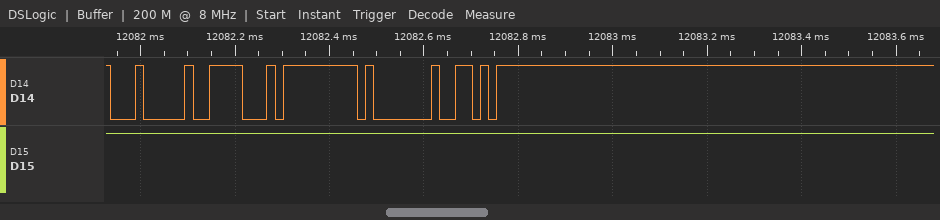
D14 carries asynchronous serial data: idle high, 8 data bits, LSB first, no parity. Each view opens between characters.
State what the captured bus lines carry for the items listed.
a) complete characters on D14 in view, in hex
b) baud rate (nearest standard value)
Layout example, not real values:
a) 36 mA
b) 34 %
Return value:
a) 04, 1E, FF, 01, D6
b) 57600 baud
